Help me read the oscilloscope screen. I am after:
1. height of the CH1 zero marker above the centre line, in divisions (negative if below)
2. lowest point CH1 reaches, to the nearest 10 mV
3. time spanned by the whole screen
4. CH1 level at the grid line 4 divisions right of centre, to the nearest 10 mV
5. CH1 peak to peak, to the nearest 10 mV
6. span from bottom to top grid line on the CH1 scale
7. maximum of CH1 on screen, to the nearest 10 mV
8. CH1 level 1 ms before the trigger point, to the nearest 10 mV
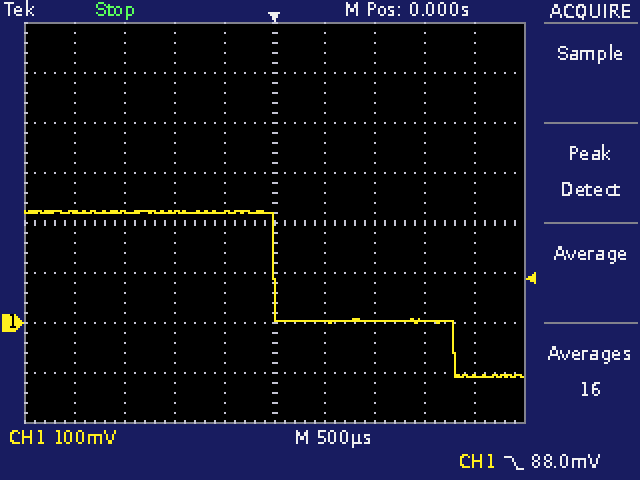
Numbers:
-2.0 div
-110 mV
5 ms
-110 mV
330 mV
800 mV
220 mV
220 mV
